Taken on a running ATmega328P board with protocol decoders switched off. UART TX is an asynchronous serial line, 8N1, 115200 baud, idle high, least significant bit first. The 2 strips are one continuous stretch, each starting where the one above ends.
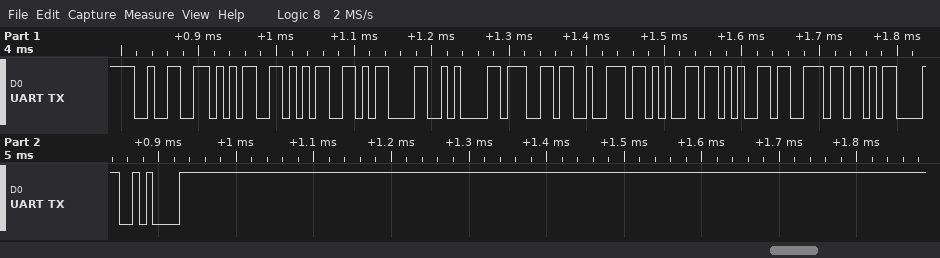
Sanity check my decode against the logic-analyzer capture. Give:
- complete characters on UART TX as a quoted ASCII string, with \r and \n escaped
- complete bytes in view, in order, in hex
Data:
"255\r\ngreen\r\n"
32 35 35 0D 0A 67 72 65 65 6E 0D 0A
